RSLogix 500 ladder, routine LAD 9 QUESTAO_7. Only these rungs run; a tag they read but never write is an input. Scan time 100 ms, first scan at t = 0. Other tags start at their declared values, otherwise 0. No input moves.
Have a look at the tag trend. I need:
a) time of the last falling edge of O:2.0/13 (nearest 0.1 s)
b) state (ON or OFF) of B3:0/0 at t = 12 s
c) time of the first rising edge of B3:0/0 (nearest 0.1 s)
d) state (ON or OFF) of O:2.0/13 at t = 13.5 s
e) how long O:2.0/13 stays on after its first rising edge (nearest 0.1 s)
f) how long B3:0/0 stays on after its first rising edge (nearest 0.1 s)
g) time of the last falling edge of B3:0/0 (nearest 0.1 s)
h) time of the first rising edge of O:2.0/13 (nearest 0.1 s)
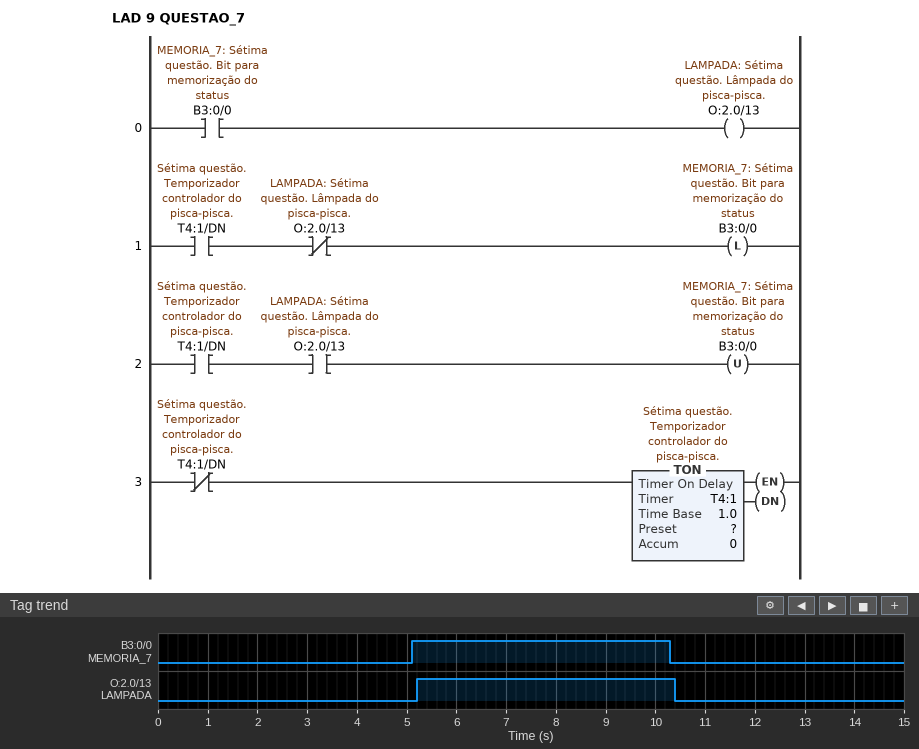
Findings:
10.4 s
OFF
5.1 s
OFF
5.2 s
5.2 s
10.3 s
5.2 s
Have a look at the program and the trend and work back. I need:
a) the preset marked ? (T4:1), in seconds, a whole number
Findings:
5 s
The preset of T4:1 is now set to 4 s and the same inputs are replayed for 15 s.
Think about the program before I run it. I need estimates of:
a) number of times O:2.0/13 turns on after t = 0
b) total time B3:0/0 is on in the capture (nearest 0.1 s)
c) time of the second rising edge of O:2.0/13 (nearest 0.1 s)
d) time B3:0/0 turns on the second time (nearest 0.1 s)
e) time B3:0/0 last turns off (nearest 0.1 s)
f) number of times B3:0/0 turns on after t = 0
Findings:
2
6.7 s
12.6 s
12.5 s
8.3 s
2
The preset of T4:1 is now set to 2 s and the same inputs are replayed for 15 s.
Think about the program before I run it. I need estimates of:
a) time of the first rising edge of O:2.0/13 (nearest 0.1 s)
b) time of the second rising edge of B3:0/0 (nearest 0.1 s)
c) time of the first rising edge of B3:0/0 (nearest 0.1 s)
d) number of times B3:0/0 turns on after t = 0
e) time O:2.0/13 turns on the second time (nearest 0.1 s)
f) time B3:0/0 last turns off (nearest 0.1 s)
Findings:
2.2 s
6.5 s
2.1 s
3
6.6 s
13.1 s
